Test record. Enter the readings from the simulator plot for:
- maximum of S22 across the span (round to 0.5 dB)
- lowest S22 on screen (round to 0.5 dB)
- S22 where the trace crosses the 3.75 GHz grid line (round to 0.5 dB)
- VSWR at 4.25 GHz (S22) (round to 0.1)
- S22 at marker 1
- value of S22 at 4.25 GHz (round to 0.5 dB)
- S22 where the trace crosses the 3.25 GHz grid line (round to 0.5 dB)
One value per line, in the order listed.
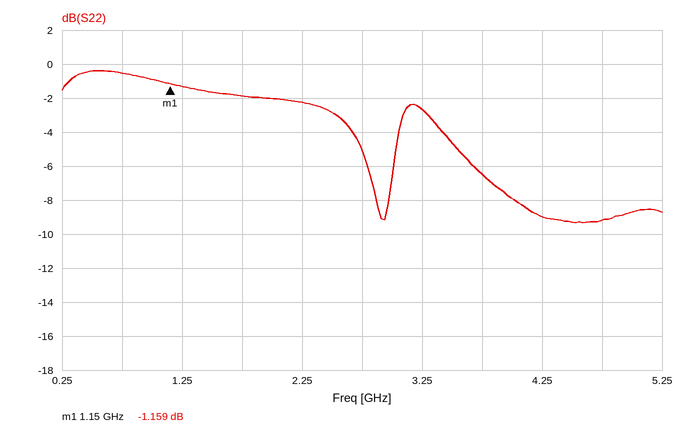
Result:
-0.5 dB
-9.5 dB
-6.5 dB
2.1
-1.159 dB
-9.0 dB
-2.5 dB
